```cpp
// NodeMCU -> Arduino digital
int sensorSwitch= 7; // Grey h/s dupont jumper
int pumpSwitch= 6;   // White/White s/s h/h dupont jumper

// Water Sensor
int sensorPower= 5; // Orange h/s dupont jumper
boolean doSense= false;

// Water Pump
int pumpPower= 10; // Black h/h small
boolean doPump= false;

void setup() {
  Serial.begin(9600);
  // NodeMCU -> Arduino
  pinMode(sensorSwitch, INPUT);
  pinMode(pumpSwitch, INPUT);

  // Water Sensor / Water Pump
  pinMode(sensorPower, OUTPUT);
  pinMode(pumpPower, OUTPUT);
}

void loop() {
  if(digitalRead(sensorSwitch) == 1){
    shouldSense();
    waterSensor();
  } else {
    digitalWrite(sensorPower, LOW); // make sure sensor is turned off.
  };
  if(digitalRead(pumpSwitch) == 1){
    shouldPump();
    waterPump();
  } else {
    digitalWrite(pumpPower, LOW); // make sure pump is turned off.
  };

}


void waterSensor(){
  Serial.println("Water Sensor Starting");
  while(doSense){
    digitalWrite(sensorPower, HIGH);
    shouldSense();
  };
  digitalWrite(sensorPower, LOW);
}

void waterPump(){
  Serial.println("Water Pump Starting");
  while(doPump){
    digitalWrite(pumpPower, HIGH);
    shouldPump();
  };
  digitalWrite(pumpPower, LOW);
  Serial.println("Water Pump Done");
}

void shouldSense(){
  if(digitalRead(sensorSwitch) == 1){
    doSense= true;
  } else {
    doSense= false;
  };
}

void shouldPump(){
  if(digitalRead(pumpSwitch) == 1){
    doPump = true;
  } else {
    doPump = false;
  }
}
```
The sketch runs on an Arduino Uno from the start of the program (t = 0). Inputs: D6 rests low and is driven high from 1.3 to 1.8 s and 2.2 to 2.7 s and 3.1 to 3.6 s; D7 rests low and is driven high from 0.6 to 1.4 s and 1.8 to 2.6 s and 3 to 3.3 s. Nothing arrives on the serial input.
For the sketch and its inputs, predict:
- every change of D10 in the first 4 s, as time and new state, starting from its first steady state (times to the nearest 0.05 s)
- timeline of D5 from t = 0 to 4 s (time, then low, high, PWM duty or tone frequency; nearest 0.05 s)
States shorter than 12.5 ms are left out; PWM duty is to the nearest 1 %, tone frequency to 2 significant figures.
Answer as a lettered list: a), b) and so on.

a) 0 s low; 1.4 s high; 1.8 s low; 2.6 s high; 2.7 s low; 3.3 s high; 3.6 s low
b) 0 s low; 0.6 s high; 1.4 s low; 1.8 s high; 2.6 s low; 3 s high; 3.3 s low
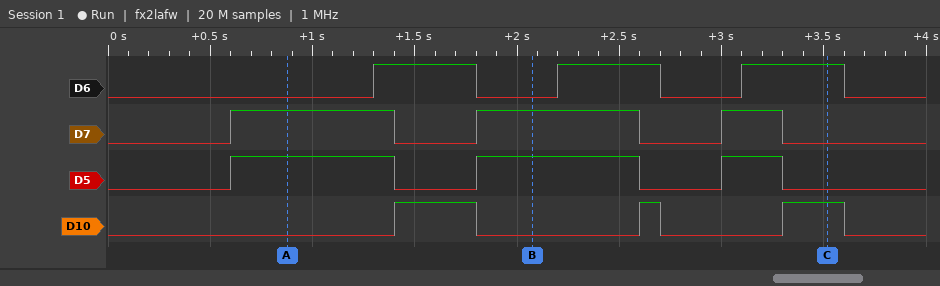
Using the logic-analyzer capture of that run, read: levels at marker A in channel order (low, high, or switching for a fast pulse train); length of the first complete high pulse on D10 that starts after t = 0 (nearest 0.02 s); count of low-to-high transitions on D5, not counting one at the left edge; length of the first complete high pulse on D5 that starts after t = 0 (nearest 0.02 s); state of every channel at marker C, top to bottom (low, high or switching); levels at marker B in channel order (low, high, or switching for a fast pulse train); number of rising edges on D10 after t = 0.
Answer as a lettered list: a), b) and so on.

a) D6 low, D7 high, D5 high, D10 low
b) 0.40 s
c) 3
d) 0.80 s
e) D6 high, D7 low, D5 low, D10 high
f) D6 low, D7 high, D5 high, D10 low
g) 3
